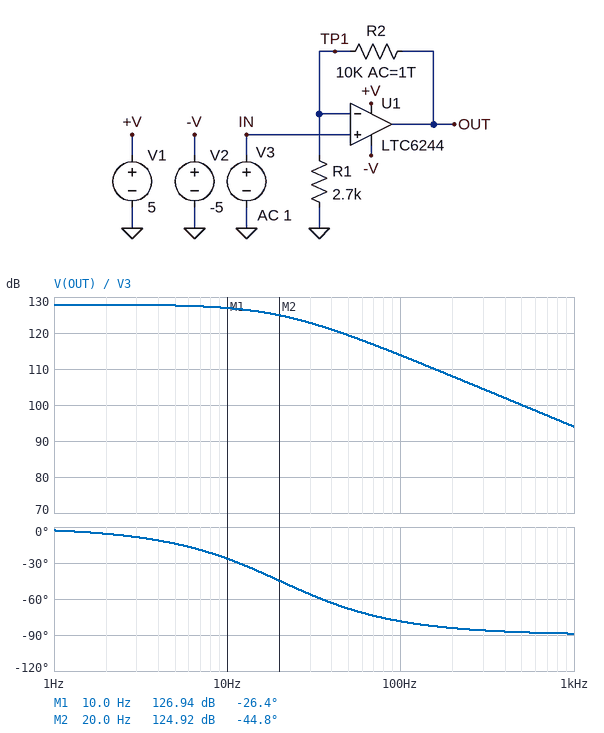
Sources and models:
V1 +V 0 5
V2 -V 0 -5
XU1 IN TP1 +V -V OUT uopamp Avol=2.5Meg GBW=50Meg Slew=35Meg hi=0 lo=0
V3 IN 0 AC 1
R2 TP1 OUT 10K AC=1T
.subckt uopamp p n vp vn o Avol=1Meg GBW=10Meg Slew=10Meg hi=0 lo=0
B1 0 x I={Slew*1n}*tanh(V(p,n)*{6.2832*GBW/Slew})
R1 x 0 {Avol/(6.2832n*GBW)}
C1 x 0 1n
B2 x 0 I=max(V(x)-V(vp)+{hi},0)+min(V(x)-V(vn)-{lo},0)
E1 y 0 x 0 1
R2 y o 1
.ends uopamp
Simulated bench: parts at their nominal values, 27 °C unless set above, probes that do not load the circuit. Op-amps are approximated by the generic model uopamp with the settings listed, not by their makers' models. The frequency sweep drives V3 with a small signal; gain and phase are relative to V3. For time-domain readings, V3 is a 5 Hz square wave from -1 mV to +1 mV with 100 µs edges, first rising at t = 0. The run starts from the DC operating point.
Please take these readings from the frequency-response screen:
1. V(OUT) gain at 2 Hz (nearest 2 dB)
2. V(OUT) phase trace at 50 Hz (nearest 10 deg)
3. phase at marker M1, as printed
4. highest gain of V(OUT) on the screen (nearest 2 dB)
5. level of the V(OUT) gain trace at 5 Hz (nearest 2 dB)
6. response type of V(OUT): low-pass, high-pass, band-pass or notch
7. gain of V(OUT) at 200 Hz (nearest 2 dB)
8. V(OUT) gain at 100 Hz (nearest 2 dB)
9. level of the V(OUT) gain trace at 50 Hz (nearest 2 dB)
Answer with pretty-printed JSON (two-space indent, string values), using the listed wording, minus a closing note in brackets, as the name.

{
  "V(OUT) gain at 2 Hz": "128 dB",
  "V(OUT) phase trace at 50 Hz": "-70 deg",
  "phase at marker M1, as printed": "-26.4 deg",
  "highest gain of V(OUT) on the screen": "128 dB",
  "level of the V(OUT) gain trace at 5 Hz": "128 dB",
  "response type of V(OUT): low-pass, high-pass, band-pass or notch": "low-pass",
  "gain of V(OUT) at 200 Hz": "108 dB",
  "V(OUT) gain at 100 Hz": "114 dB",
  "level of the V(OUT) gain trace at 50 Hz": "120 dB"
}
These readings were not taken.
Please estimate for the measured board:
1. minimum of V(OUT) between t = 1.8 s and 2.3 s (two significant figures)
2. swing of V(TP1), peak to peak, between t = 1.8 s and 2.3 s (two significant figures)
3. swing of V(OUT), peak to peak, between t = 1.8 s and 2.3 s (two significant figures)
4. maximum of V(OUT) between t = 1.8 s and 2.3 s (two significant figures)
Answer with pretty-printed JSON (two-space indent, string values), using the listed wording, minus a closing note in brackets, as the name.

{
  "minimum of V(OUT) between t = 1.8 s and 2.3 s": "-4.7 mV",
  "swing of V(TP1), peak to peak, between t = 1.8 s and 2.3 s": "2.0 mV",
  "swing of V(OUT), peak to peak, between t = 1.8 s and 2.3 s": "9.4 mV",
  "maximum of V(OUT) between t = 1.8 s and 2.3 s": "4.7 mV"
}
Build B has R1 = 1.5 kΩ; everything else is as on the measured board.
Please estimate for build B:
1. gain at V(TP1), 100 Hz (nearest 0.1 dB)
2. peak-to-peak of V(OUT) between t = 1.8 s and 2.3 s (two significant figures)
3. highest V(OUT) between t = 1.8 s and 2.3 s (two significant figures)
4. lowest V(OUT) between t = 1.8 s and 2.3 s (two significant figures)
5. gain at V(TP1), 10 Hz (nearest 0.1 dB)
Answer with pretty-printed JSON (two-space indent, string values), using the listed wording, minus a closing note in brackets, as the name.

{
  "gain at V(TP1), 100 Hz": "-62.7 dB",
  "peak-to-peak of V(OUT) between t = 1.8 s and 2.3 s": "15 mV",
  "highest V(OUT) between t = 1.8 s and 2.3 s": "7.7 mV",
  "lowest V(OUT) between t = 1.8 s and 2.3 s": "-7.7 mV",
  "gain at V(TP1), 10 Hz": "-49.5 dB"
}
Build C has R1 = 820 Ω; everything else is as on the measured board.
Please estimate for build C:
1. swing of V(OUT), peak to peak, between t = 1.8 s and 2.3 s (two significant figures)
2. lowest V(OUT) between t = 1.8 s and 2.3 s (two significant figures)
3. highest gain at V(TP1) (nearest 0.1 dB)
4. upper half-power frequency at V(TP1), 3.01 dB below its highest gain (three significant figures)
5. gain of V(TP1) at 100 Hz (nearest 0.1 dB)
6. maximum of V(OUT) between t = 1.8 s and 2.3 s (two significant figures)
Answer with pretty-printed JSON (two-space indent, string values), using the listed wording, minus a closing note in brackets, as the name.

{
  "swing of V(OUT), peak to peak, between t = 1.8 s and 2.3 s": "26 mV",
  "lowest V(OUT) between t = 1.8 s and 2.3 s": "-13 mV",
  "highest gain at V(TP1)": "-53.8 dB",
  "upper half-power frequency at V(TP1), 3.01 dB below its highest gain": "20.0 Hz",
  "gain of V(TP1) at 100 Hz": "-67.9 dB",
  "maximum of V(OUT) between t = 1.8 s and 2.3 s": "13 mV"
}
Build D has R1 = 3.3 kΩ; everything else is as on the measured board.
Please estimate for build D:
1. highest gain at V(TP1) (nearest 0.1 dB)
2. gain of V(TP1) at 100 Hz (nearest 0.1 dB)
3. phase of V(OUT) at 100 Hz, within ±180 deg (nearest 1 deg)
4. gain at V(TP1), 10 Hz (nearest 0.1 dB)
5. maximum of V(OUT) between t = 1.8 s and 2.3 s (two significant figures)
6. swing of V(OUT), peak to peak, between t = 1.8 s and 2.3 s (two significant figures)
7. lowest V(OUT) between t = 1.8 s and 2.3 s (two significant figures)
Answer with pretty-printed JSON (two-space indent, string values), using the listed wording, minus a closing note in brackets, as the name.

{
  "highest gain at V(TP1)": "-41.7 dB",
  "gain of V(TP1) at 100 Hz": "-55.8 dB",
  "phase of V(OUT) at 100 Hz, within ±180 deg": "-79 deg",
  "gain at V(TP1), 10 Hz": "-42.7 dB",
  "maximum of V(OUT) between t = 1.8 s and 2.3 s": "4.0 mV",
  "swing of V(OUT), peak to peak, between t = 1.8 s and 2.3 s": "8.1 mV",
  "lowest V(OUT) between t = 1.8 s and 2.3 s": "-4.0 mV"
}
